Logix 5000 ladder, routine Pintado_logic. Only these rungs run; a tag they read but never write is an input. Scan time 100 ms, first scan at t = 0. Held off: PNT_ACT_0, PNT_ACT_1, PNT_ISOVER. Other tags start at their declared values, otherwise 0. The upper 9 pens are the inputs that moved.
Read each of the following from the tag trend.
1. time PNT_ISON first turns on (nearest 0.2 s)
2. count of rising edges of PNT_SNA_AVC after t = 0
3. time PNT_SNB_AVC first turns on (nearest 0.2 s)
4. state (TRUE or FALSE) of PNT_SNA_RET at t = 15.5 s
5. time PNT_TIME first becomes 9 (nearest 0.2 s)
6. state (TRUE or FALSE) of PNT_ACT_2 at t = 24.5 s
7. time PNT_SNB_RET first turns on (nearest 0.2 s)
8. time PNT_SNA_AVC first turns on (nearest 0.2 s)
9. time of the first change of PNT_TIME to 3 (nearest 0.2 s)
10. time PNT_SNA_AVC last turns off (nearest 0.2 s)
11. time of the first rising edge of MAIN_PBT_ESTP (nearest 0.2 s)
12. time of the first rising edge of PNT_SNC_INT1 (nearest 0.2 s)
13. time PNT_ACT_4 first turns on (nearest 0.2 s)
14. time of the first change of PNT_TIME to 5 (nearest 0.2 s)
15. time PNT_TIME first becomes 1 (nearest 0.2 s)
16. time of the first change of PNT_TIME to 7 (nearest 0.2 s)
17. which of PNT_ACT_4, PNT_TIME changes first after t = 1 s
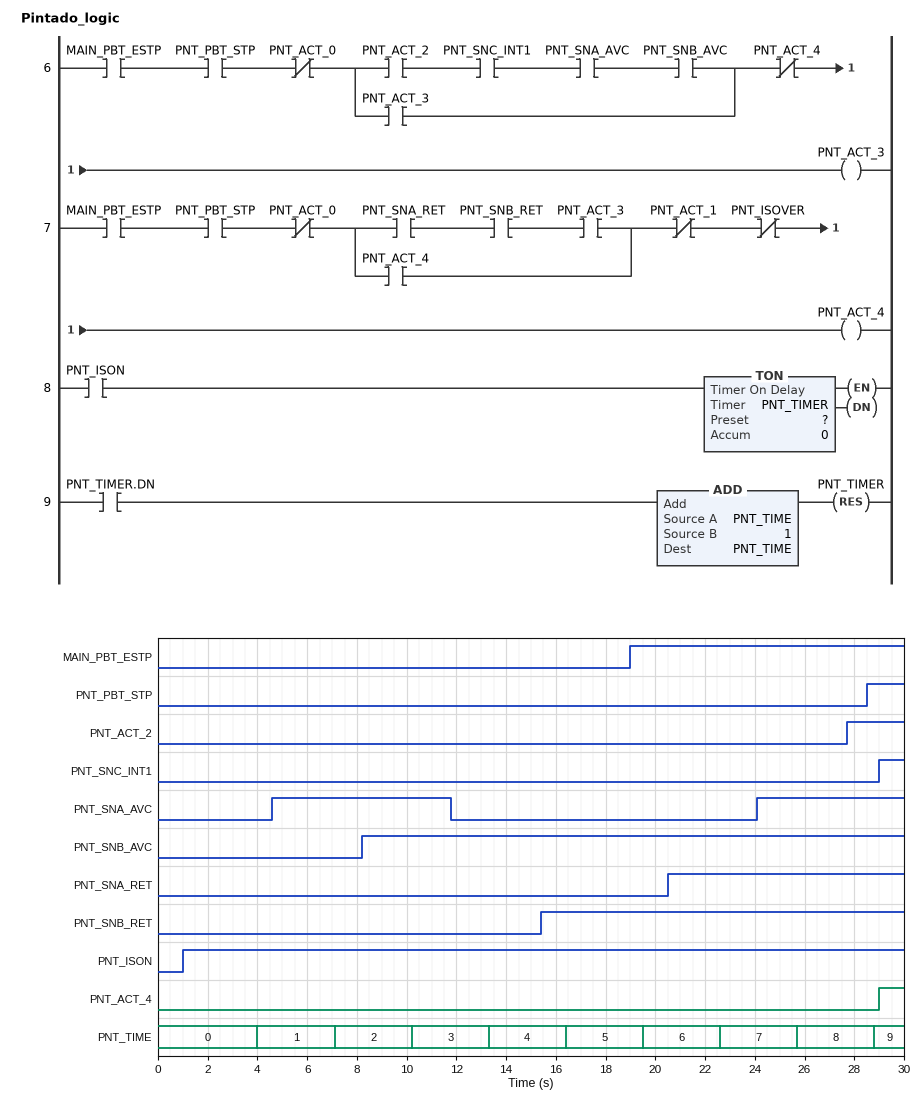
1.0 s
2
8.2 s
FALSE
28.8 s
FALSE
15.4 s
4.6 s
10.2 s
11.8 s
19.0 s
29.0 s
29.0 s
16.4 s
4.0 s
22.6 s
PNT_TIME
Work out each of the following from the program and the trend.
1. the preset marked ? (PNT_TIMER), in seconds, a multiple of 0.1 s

3.0 s
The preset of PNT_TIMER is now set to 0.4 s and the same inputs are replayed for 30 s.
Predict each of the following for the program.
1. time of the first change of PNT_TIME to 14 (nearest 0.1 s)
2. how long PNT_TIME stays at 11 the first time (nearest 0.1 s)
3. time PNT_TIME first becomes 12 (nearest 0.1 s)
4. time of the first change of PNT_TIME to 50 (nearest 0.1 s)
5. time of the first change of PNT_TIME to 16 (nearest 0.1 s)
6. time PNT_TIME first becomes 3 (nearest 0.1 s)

7.9 s
0.5 s
6.9 s
25.9 s
8.9 s
2.4 s
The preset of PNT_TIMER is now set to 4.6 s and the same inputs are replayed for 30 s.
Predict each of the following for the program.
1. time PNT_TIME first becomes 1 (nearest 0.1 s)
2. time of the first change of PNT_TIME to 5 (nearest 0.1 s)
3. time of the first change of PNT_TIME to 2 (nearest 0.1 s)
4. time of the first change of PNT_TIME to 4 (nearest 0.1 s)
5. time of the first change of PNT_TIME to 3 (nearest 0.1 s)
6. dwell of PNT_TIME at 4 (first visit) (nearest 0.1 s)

5.6 s
24.4 s
10.3 s
19.7 s
15.0 s
4.7 s
